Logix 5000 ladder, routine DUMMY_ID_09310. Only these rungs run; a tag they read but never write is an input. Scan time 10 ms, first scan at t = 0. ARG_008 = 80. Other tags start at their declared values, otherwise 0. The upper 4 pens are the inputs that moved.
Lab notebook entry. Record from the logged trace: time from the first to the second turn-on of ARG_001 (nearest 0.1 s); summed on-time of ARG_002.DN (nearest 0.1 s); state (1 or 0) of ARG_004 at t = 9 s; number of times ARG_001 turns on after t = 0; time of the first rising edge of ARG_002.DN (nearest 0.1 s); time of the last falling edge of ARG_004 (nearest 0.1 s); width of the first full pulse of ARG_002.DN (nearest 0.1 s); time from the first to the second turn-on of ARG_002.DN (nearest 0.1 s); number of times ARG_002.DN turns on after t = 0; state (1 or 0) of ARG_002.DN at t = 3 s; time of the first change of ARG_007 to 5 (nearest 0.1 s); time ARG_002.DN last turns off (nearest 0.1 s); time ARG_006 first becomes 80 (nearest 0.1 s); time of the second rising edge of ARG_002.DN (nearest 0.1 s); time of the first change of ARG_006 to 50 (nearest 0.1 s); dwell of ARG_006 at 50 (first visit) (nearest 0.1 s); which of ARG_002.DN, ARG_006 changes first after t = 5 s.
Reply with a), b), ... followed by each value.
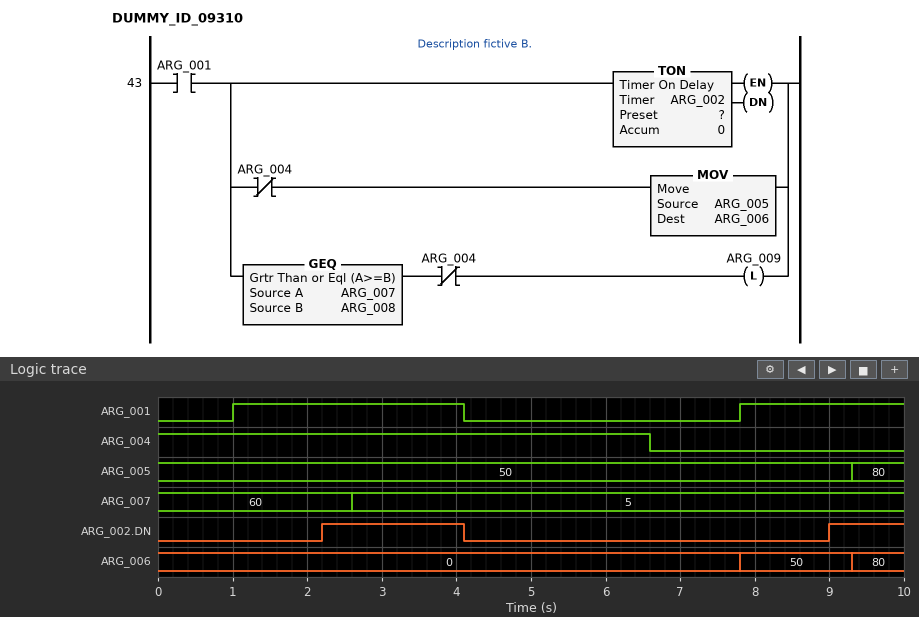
a) 6.8 s
b) 2.9 s
c) 0
d) 2
e) 2.2 s
f) 6.6 s
g) 1.9 s
h) 6.8 s
i) 2
j) 1
k) 2.6 s
l) 4.1 s
m) 9.3 s
n) 9.0 s
o) 7.8 s
p) 1.5 s
q) ARG_006
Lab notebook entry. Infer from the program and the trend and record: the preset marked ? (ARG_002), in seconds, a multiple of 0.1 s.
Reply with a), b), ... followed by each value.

a) 1.2 s
